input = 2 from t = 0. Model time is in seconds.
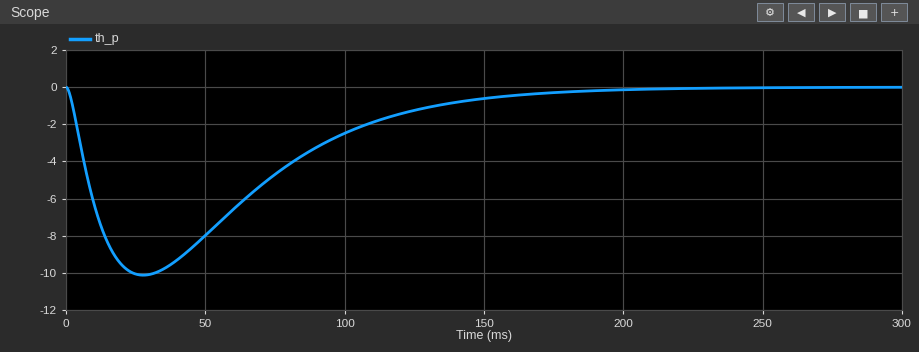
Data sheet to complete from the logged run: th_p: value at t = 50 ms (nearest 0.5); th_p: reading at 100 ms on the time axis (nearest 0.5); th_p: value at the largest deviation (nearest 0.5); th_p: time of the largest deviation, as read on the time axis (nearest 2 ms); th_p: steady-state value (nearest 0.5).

-8.0
-2.5
-10.0
28 ms
0.0
